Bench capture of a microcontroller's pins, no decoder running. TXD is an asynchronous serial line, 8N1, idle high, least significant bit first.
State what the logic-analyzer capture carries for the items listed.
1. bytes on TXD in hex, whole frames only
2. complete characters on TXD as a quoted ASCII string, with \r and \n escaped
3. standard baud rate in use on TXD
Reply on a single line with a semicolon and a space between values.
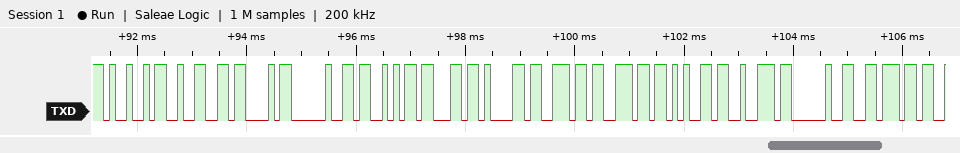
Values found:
49 32 43 20 53 63 61 6E 6E 65 72 20 76; "I2C Scanner v"; 9600 baud
